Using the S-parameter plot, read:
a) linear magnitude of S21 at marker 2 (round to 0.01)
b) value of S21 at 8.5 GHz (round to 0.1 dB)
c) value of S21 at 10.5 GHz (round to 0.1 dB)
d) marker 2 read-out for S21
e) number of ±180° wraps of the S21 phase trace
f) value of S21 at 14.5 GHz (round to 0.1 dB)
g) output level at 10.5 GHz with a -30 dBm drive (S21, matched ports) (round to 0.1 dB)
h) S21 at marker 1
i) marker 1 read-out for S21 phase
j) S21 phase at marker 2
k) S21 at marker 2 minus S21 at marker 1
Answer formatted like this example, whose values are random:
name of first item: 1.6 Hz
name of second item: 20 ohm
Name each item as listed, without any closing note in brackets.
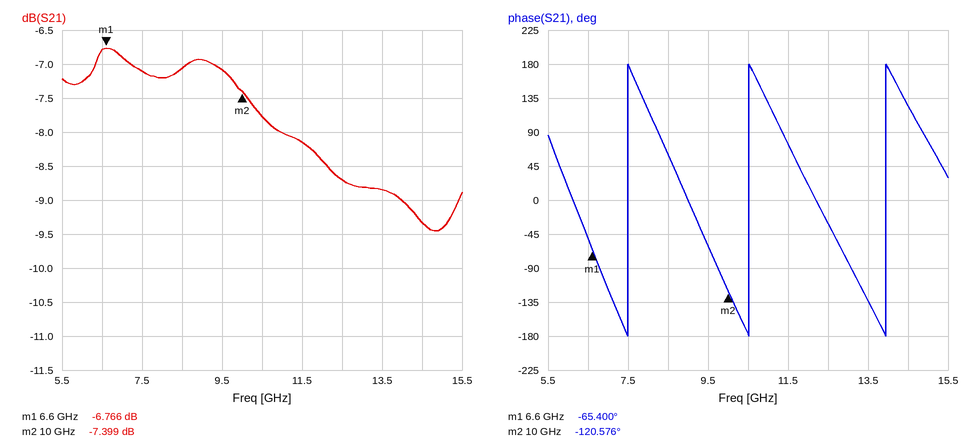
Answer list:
linear magnitude of S21 at marker 2: 0.43
value of S21 at 8.5 GHz: -7.1 dB
value of S21 at 10.5 GHz: -7.8 dB
marker 2 read-out for S21: -7.399 dB
number of ±180° wraps of the S21 phase trace: 3
value of S21 at 14.5 GHz: -9.3 dB
output level at 10.5 GHz with a -30 dBm drive (S21, matched ports): -37.8 dBm
S21 at marker 1: -6.766 dB
marker 1 read-out for S21 phase: -65.400°
S21 phase at marker 2: -120.576°
S21 at marker 2 minus S21 at marker 1: -0.633 dB
